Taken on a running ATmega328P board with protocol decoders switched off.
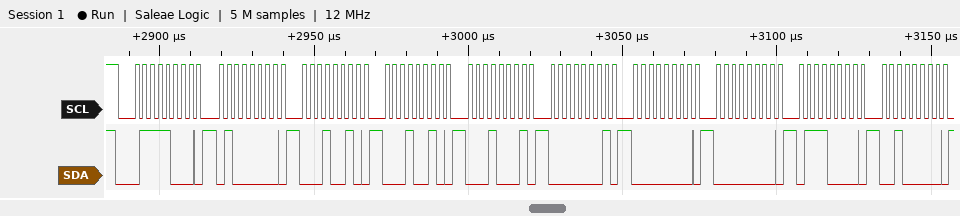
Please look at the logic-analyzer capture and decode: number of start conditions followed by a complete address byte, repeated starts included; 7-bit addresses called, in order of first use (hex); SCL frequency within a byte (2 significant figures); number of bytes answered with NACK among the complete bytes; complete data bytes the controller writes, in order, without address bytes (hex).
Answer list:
1
0x3C
400 kHz
0
40 12 12 11 01 00 00 70 20
